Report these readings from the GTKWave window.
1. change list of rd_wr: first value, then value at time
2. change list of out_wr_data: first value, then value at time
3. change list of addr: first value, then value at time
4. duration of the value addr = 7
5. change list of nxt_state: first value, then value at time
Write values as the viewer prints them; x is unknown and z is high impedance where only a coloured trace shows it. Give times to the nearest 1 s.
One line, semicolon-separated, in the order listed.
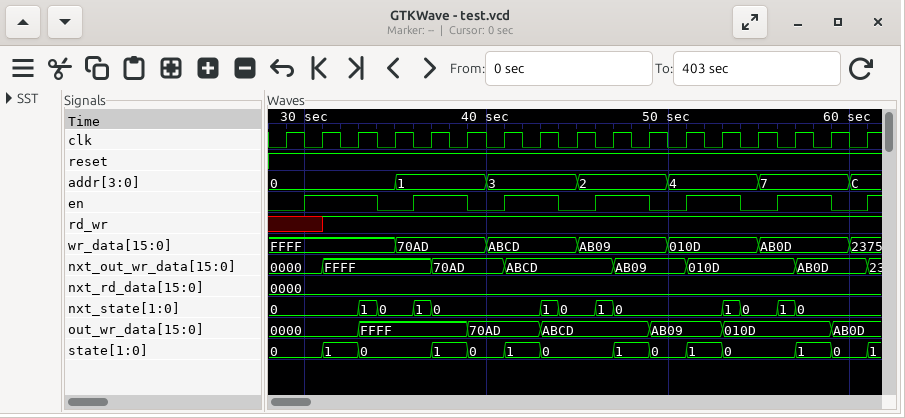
x, 1 at 31 s; 0000, FFFF at 33 s, 70AD at 39 s, ABCD at 43 s, AB09 at 49 s, 010D at 53 s, AB0D at 59 s; 0, 1 at 35 s, 3 at 40 s, 2 at 45 s, 4 at 50 s, 7 at 55 s, C at 60 s; 5 s; 0, 1 at 33 s, 0 at 34 s, 1 at 36 s, 0 at 37 s, 1 at 43 s, 0 at 44 s, 1 at 46 s, 0 at 47 s, 1 at 53 s, 0 at 54 s, 1 at 56 s, 0 at 57 s
